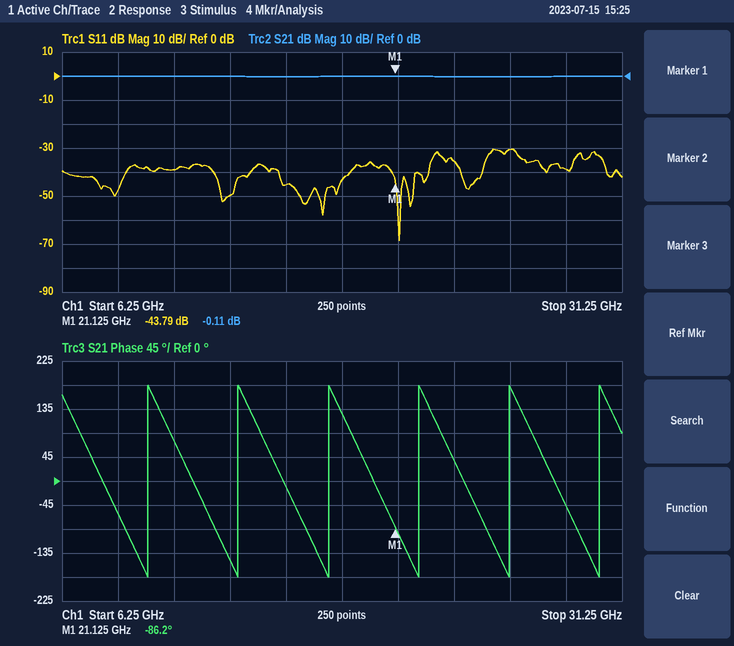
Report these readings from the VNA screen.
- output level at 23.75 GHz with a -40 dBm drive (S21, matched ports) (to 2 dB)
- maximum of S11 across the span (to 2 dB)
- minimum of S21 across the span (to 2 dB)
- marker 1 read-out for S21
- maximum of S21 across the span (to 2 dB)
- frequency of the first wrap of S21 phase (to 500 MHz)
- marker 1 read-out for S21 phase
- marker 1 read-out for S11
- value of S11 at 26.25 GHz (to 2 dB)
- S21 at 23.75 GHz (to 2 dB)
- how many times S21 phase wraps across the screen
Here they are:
-40 dBm
-30 dB
0 dB
-0.11 dB
0 dB
10.0 GHz
-86.2°
-43.79 dB
-30 dB
0 dB
6
